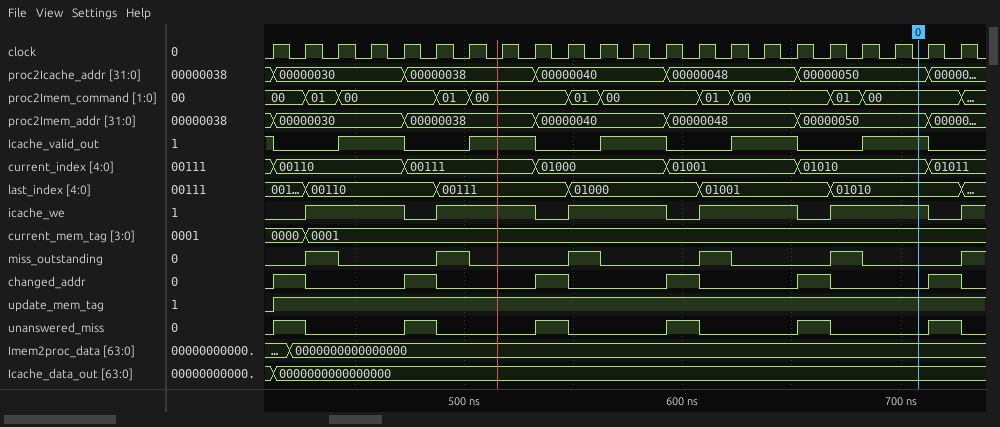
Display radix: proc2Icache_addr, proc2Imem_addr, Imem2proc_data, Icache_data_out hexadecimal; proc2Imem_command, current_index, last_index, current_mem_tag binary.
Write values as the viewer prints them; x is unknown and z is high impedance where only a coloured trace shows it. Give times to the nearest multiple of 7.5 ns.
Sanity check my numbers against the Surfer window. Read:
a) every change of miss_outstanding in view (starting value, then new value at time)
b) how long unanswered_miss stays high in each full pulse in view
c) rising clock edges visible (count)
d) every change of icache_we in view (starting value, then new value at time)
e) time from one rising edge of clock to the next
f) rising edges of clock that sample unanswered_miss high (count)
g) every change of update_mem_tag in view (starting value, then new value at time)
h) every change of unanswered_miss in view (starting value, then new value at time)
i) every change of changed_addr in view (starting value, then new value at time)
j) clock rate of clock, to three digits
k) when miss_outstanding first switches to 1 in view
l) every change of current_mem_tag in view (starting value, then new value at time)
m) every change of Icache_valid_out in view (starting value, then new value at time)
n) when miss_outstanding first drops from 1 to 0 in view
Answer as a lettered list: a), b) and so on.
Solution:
a) 0, 1 at 427.5 ns, 0 at 442.5 ns, 1 at 487.5 ns, 0 at 502.5 ns, 1 at 547.5 ns, 0 at 562.5 ns, 1 at 607.5 ns, 0 at 622.5 ns, 1 at 667.5 ns, 0 at 682.5 ns, 1 at 727.5 ns
b) 15 ns, 15 ns, 15 ns, 15 ns, 15 ns, 15 ns
c) 22
d) 0, 1 at 427.5 ns, 0 at 472.5 ns, 1 at 487.5 ns, 0 at 532.5 ns, 1 at 547.5 ns, 0 at 592.5 ns, 1 at 607.5 ns, 0 at 652.5 ns, 1 at 667.5 ns, 0 at 712.5 ns, 1 at 727.5 ns
e) 15 ns
f) 6
g) 0, 1 at 412.5 ns
h) 0, 1 at 412.5 ns, 0 at 427.5 ns, 1 at 472.5 ns, 0 at 487.5 ns, 1 at 532.5 ns, 0 at 547.5 ns, 1 at 592.5 ns, 0 at 607.5 ns, 1 at 652.5 ns, 0 at 667.5 ns, 1 at 712.5 ns, 0 at 727.5 ns
i) 0, 1 at 412.5 ns, 0 at 427.5 ns, 1 at 472.5 ns, 0 at 487.5 ns, 1 at 532.5 ns, 0 at 547.5 ns, 1 at 592.5 ns, 0 at 607.5 ns, 1 at 652.5 ns, 0 at 667.5 ns, 1 at 712.5 ns, 0 at 727.5 ns
j) 66.7 MHz
k) 427.5 ns
l) 0000, 0001 at 427.5 ns
m) 1, 0 at 412.5 ns, 1 at 442.5 ns, 0 at 472.5 ns, 1 at 502.5 ns, 0 at 532.5 ns, 1 at 562.5 ns, 0 at 592.5 ns, 1 at 622.5 ns, 0 at 652.5 ns, 1 at 682.5 ns, 0 at 712.5 ns
n) 442.5 ns
